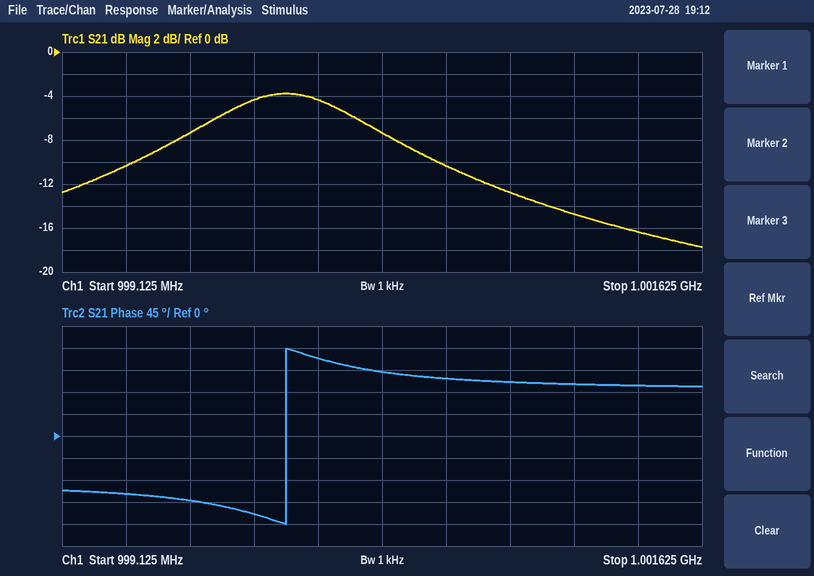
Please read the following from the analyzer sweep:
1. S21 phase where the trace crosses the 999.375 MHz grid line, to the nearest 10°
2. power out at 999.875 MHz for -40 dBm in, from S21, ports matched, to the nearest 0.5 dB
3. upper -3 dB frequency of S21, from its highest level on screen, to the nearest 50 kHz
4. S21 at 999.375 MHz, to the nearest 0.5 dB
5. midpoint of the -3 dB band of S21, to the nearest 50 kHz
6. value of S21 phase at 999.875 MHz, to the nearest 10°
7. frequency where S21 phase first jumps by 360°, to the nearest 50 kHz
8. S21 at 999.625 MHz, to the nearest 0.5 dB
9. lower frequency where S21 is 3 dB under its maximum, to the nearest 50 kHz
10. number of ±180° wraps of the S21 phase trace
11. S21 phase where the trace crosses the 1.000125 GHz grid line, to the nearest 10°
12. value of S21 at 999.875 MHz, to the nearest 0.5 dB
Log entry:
-120°
-44.5 dBm
1.00035 GHz
-10.5 dB
1.00000 GHz
-160°
1.00000 GHz
-7.5 dB
999.65 MHz
1
160°
-4.5 dB
